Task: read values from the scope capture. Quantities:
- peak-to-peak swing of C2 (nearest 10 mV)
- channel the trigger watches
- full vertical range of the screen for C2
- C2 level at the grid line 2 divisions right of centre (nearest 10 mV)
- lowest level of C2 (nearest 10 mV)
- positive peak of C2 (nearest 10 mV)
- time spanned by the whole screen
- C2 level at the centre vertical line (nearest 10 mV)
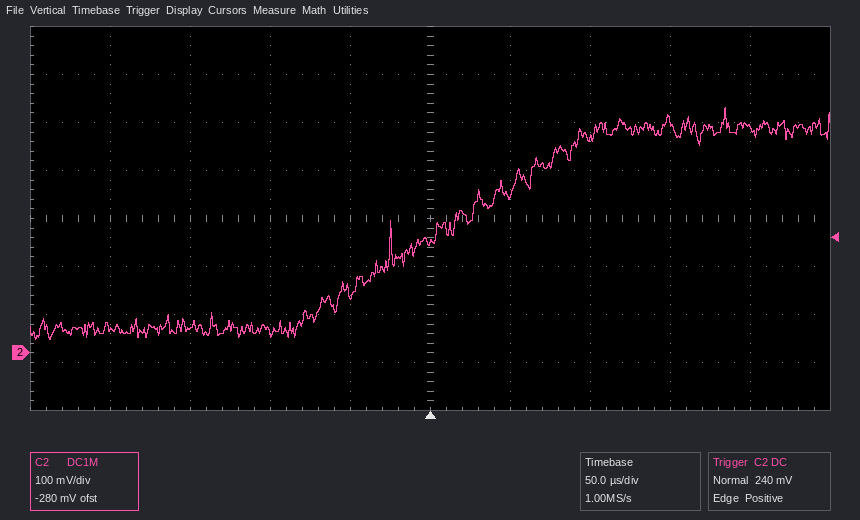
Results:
480 mV
C2
800 mV
450 mV
30 mV
510 mV
500 µs
230 mV
